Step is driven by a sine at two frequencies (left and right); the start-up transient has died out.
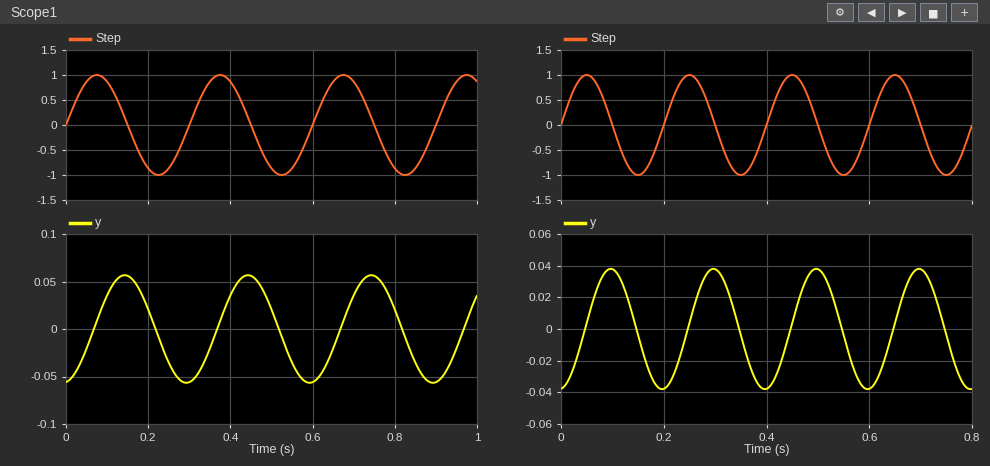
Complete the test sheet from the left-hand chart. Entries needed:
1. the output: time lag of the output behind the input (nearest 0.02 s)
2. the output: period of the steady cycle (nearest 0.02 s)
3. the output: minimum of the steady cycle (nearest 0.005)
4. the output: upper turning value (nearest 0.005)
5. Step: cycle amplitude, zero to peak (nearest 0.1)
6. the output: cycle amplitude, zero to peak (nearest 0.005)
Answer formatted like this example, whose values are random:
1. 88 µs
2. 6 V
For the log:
1. 0.06 s
2. 0.30 s
3. -0.055
4. 0.055
5. 1.0
6. 0.055
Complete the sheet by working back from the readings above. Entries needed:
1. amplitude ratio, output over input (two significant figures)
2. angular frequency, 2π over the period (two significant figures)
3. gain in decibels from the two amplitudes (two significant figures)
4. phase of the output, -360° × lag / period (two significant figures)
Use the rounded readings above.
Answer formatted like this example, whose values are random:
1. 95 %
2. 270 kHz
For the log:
1. 0.055
2. 21 rad/s
3. -25 dB
4. -72°
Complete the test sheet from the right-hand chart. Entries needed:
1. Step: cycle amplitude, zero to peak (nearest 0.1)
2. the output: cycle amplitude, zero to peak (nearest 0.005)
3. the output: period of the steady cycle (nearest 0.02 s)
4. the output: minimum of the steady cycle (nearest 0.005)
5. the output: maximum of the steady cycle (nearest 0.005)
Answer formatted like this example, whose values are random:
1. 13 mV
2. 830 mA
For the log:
1. 1.0
2. 0.040
3. 0.20 s
4. -0.040
5. 0.040
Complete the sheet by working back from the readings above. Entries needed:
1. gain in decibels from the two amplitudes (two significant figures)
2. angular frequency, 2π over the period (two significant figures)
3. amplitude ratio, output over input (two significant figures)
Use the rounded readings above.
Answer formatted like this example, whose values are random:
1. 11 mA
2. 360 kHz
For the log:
1. -28 dB
2. 31 rad/s
3. 0.040
